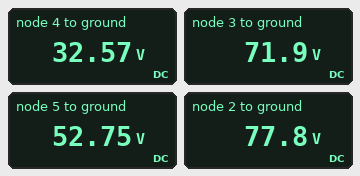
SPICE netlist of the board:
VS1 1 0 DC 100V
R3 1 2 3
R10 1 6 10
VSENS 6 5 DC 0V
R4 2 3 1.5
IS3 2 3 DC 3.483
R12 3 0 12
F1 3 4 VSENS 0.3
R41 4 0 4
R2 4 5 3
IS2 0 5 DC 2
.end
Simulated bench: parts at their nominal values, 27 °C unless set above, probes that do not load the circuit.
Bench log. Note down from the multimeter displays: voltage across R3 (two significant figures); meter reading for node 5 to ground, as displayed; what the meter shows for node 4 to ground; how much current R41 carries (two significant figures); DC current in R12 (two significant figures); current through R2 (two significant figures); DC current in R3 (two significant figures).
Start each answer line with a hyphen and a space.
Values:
- 22 V
- 52.75 V
- 32.57 V
- 8.1 A
- 6.0 A
- 6.7 A
- 7.4 A
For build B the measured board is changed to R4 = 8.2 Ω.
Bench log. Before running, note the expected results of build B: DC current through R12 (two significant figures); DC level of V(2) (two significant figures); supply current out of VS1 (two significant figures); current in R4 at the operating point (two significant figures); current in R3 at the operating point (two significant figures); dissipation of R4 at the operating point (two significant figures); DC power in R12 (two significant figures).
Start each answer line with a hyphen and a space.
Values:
- 4.9 A
- 81 V
- 11 A
- 2.8 A
- 6.3 A
- 64 W
- 280 W
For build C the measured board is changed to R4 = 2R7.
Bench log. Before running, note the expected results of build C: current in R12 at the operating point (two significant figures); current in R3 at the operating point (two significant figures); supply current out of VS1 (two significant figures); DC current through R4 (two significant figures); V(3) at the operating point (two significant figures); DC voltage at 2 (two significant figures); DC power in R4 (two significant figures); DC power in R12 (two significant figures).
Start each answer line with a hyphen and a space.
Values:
- 5.7 A
- 7.1 A
- 12 A
- 3.7 A
- 69 V
- 79 V
- 36 W
- 390 W
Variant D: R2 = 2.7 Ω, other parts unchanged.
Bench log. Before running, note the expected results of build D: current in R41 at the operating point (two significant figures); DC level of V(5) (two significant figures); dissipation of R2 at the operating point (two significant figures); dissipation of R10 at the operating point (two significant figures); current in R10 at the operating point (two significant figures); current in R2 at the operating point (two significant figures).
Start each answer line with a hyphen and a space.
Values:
- 8.3 A
- 52 V
- 130 W
- 230 W
- 4.8 A
- 6.8 A
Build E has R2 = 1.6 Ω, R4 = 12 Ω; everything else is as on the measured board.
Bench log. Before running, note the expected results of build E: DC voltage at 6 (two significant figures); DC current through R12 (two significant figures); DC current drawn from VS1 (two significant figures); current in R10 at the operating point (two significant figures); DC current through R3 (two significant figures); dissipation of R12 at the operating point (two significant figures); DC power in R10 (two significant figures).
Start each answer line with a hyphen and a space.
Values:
- 47 V
- 4.4 A
- 11 A
- 5.3 A
- 6.0 A
- 230 W
- 280 W
